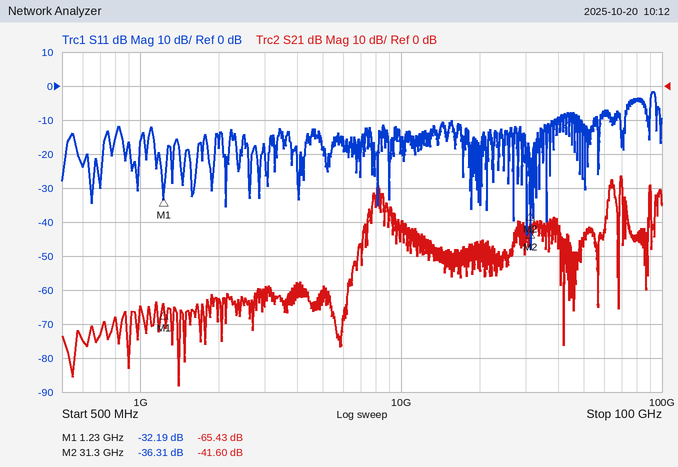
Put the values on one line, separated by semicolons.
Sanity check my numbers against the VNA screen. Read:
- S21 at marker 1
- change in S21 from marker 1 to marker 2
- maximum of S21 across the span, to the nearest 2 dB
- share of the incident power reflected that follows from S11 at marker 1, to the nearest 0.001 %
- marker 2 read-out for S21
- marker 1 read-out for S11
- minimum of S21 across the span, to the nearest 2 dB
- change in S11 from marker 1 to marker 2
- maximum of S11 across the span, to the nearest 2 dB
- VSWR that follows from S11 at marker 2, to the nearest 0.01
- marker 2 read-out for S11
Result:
-65.43 dB; 23.83 dB; -26 dB; 0.060 %; -41.60 dB; -32.19 dB; -88 dB; -4.12 dB; -2 dB; 1.03; -36.31 dB
